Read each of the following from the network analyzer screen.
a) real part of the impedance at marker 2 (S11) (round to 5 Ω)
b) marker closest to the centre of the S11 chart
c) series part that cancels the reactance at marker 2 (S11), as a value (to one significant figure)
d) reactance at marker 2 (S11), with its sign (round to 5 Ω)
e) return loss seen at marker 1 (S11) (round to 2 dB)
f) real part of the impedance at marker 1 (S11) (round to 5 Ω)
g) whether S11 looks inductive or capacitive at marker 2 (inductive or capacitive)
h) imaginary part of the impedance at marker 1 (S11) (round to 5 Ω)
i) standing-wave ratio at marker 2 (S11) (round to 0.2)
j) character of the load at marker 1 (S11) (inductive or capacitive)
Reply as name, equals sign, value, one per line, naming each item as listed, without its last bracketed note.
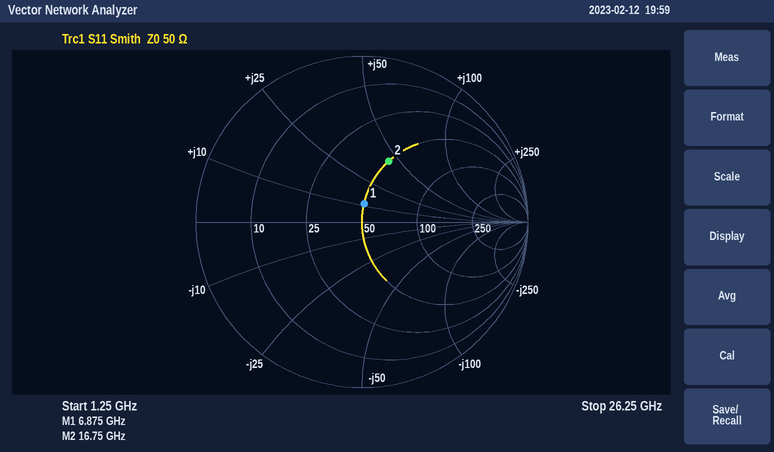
real part of the impedance at marker 2 (S11) = 50 Ω
marker closest to the centre of the S11 chart = marker 1
series part that cancels the reactance at marker 2 (S11), as a value = 200 fF
reactance at marker 2 (S11), with its sign = +45 Ω
return loss seen at marker 1 (S11) = 20 dB
real part of the impedance at marker 1 (S11) = 50 Ω
whether S11 looks inductive or capacitive at marker 2 = inductive
imaginary part of the impedance at marker 1 (S11) = +10 Ω
standing-wave ratio at marker 2 (S11) = 2.4
character of the load at marker 1 (S11) = inductive
